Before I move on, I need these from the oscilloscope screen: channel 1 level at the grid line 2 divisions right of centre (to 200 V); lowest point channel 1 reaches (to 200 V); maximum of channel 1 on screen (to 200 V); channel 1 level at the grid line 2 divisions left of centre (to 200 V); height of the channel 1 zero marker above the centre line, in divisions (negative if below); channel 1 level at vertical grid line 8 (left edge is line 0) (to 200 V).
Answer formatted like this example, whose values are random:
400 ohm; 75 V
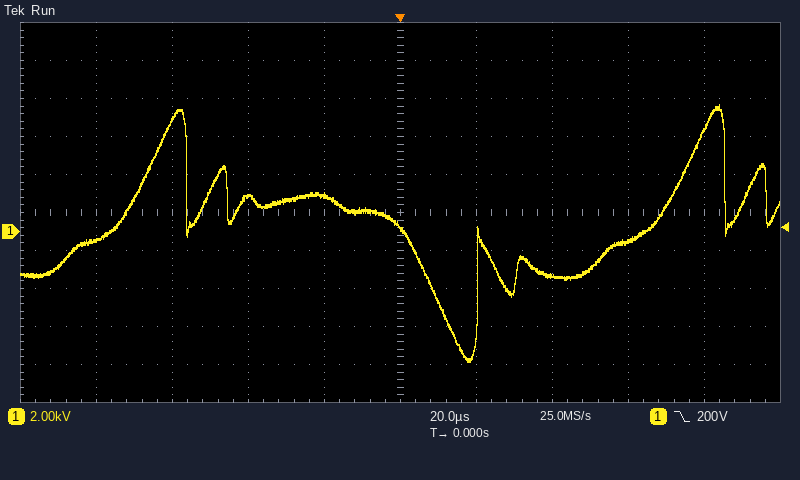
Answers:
-2.4 kV; -6.8 kV; 6.6 kV; 1.8 kV; -0.5 div; -600 V
